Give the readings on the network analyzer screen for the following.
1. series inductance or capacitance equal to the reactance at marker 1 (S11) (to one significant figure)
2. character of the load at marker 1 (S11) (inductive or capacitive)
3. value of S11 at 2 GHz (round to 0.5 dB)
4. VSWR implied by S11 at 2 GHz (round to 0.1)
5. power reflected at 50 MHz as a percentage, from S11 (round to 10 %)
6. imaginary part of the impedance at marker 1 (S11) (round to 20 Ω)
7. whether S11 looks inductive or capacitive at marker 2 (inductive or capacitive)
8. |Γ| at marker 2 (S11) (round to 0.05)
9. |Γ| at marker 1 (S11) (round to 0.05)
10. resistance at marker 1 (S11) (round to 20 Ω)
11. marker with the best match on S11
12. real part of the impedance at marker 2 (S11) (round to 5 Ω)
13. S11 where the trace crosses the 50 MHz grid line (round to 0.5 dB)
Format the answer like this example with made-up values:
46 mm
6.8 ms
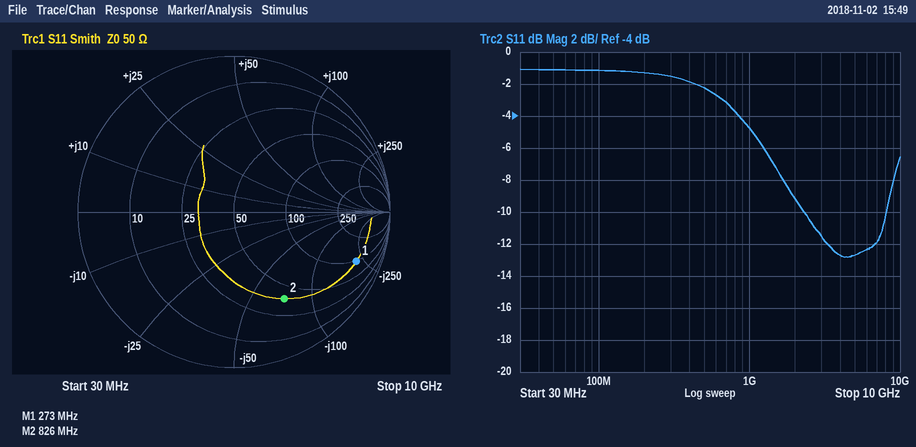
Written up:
3 pF
capacitive
-9.0 dB
2.1
80 %
-220 Ω
capacitive
0.65
0.85
100 Ω
marker 2
40 Ω
-1.0 dB
